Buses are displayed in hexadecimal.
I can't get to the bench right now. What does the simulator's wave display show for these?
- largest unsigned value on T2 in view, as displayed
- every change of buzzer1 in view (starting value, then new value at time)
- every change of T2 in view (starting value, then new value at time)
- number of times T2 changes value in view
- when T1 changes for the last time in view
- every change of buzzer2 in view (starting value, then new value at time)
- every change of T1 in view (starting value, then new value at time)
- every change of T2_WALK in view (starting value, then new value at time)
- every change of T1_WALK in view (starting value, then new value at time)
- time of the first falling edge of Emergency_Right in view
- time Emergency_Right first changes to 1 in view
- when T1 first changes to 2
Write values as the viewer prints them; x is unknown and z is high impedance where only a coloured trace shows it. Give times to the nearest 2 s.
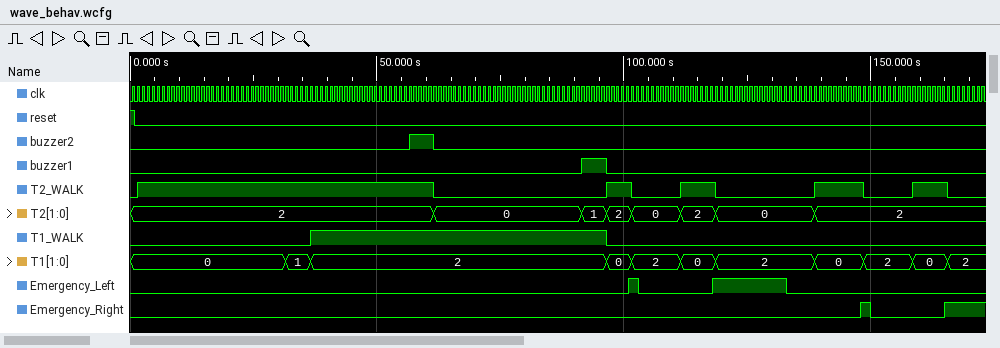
2
0, 1 at 92 s, 0 at 96 s
2, 0 at 62 s, 1 at 92 s, 2 at 96 s, 0 at 102 s, 2 at 112 s, 0 at 118 s, 2 at 138 s
7
166 s
0, 1 at 56 s, 0 at 62 s
0, 1 at 32 s, 2 at 36 s, 0 at 96 s, 2 at 102 s, 0 at 112 s, 2 at 118 s, 0 at 138 s, 2 at 148 s, 0 at 158 s, 2 at 166 s
0, 1 at 2 s, 0 at 62 s, 1 at 96 s, 0 at 102 s, 1 at 112 s, 0 at 118 s, 1 at 138 s, 0 at 148 s, 1 at 158 s, 0 at 166 s
0, 1 at 36 s, 0 at 96 s
150 s
148 s
36 s
